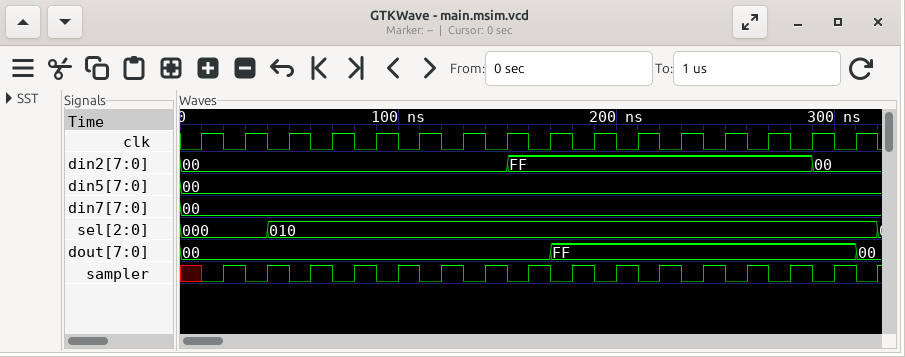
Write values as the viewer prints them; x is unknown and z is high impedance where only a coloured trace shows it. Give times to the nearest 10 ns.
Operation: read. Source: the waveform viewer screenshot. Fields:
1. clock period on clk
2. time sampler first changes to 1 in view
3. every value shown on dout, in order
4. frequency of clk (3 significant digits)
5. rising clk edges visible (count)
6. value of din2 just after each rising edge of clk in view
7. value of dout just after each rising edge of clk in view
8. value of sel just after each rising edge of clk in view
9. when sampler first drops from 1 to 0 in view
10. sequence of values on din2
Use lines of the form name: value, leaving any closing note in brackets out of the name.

clock period on clk: 20 ns
time sampler first changes to 1 in view: 20 ns
every value shown on dout, in order: 00, FF, 00
frequency of clk: 50.0 MHz
rising clk edges visible: 16
value of din2 just after each rising edge of clk in view: 00, 00, 00, 00, 00, 00, 00, FF, FF, FF, FF, FF, FF, FF, 00, 00
value of dout just after each rising edge of clk in view: 00, 00, 00, 00, 00, 00, 00, 00, FF, FF, FF, FF, FF, FF, FF, 00
value of sel just after each rising edge of clk in view: 000, 000, 010, 010, 010, 010, 010, 010, 010, 010, 010, 010, 010, 010, 010, 010
when sampler first drops from 1 to 0 in view: 30 ns
sequence of values on din2: 00, FF, 00
